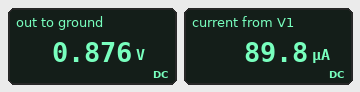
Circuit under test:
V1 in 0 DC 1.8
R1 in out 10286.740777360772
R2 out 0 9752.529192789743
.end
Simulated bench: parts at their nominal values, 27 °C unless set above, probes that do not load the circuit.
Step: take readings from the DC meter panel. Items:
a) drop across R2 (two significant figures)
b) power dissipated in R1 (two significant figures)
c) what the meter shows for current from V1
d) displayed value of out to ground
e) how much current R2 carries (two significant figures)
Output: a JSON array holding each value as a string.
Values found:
["880 mV", "83 µW", "89.8 µA", "0.876 V", "90 µA"]
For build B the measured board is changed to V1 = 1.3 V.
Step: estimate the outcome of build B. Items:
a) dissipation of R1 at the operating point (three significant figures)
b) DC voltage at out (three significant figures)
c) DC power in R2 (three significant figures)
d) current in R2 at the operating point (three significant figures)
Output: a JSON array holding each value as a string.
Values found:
["43.3 µW", "633 mV", "41.0 µW", "64.9 µA"]
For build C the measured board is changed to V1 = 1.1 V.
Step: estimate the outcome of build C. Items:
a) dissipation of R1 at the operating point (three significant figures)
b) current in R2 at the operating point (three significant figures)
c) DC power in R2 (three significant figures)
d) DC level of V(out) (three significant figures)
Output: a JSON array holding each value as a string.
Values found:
["31.0 µW", "54.9 µA", "29.4 µW", "535 mV"]
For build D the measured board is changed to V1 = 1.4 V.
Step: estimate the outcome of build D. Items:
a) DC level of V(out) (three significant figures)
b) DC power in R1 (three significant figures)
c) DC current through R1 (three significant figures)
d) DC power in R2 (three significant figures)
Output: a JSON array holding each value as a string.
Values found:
["681 mV", "50.2 µW", "69.9 µA", "47.6 µW"]
